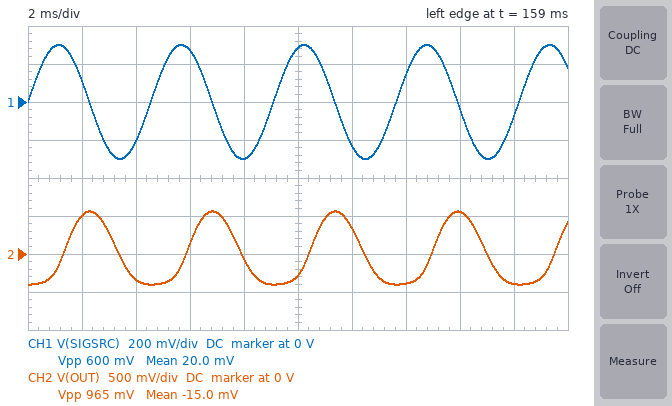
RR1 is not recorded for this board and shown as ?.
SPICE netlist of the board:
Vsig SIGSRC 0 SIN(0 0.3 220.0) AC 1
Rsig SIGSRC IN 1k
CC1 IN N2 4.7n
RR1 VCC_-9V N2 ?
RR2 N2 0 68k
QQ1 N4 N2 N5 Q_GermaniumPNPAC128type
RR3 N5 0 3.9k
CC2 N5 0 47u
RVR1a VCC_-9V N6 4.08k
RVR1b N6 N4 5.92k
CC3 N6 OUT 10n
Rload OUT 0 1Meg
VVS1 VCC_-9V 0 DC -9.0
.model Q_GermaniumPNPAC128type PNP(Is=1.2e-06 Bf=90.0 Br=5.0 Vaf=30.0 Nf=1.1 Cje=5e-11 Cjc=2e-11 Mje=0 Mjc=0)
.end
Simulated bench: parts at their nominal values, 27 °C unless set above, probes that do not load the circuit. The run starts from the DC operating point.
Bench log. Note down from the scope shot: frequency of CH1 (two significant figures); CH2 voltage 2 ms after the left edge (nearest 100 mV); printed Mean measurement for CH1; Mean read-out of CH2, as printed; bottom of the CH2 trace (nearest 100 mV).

220 Hz
500 mV
20.0 mV
-15.0 mV
-400 mV
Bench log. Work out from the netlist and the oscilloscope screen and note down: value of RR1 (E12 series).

1 MΩ
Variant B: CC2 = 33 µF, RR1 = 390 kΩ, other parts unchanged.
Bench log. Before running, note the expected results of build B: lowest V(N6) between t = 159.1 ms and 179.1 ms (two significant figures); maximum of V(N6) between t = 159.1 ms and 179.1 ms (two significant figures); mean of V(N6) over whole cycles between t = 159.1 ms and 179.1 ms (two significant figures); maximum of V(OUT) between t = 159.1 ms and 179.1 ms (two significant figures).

-8.5 V
-7.3 V
-7.9 V
630 mV
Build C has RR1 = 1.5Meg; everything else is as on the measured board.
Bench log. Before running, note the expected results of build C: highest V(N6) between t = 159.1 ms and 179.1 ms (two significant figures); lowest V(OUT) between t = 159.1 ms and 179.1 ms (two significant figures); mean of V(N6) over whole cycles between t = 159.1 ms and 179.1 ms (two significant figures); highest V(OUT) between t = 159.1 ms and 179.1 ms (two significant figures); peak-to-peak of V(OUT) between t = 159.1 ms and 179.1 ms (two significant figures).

-8.2 V
-290 mV
-8.7 V
480 mV
770 mV
